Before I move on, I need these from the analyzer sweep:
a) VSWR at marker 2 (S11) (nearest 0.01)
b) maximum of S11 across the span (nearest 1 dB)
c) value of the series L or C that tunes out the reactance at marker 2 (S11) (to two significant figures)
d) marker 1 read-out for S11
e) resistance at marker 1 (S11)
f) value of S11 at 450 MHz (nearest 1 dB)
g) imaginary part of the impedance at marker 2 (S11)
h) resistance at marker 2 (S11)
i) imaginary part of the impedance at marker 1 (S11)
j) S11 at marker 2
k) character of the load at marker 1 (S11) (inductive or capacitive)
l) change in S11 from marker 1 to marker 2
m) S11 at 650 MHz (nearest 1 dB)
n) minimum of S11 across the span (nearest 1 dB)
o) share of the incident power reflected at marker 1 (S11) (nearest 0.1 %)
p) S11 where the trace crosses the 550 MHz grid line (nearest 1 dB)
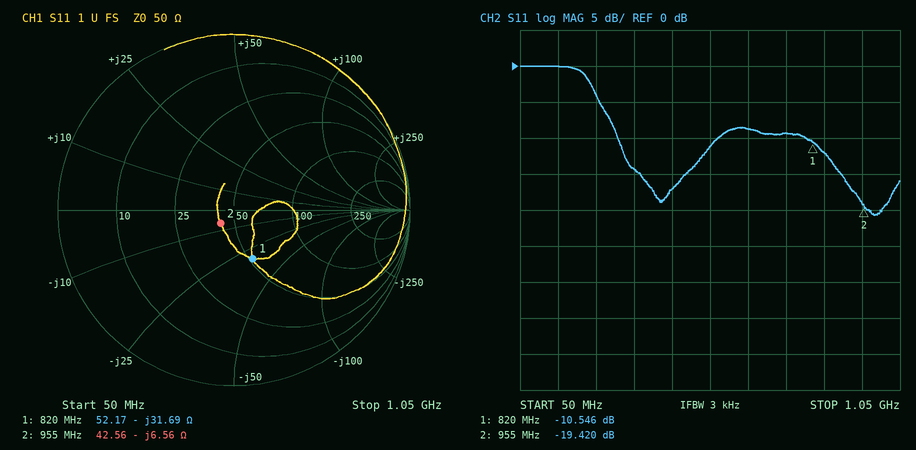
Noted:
1.24
0 dB
1.1 nH
-10.546 dB
52.17 Ω
-17 dB
-6.56 Ω
42.56 Ω
-31.69 Ω
-19.420 dB
capacitive
-8.874 dB
-9 dB
-21 dB
8.8 %
-11 dB
